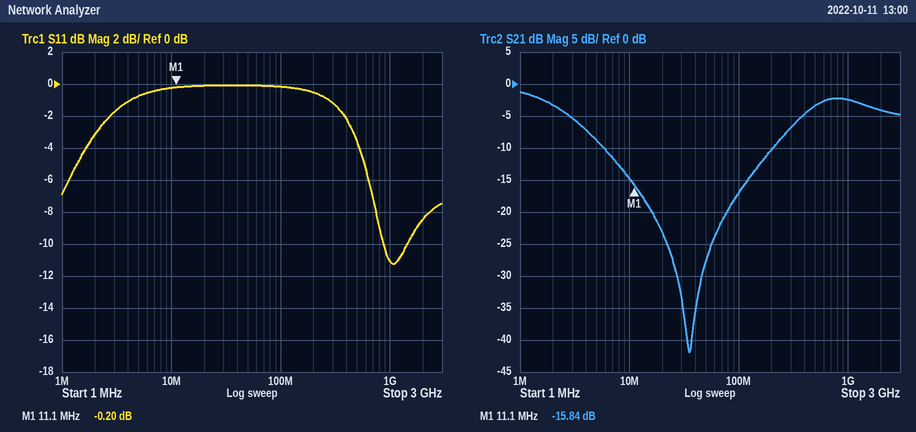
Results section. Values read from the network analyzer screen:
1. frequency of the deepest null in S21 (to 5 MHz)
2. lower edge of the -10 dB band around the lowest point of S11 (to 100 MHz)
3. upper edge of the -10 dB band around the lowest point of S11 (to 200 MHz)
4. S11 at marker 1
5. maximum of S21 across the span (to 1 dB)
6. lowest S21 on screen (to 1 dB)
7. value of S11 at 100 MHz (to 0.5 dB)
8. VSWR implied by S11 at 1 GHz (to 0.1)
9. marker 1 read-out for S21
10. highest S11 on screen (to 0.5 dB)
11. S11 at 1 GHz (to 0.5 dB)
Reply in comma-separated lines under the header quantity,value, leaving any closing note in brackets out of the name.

quantity,value
frequency of the deepest null in S21,35 MHz
lower edge of the -10 dB band around the lowest point of S11,900 MHz
upper edge of the -10 dB band around the lowest point of S11,1.4 GHz
S11 at marker 1,-0.20 dB
maximum of S21 across the span,-1 dB
lowest S21 on screen,-42 dB
value of S11 at 100 MHz,0.0 dB
VSWR implied by S11 at 1 GHz,1.8
marker 1 read-out for S21,-15.84 dB
highest S11 on screen,0.0 dB
S11 at 1 GHz,-11.0 dB
